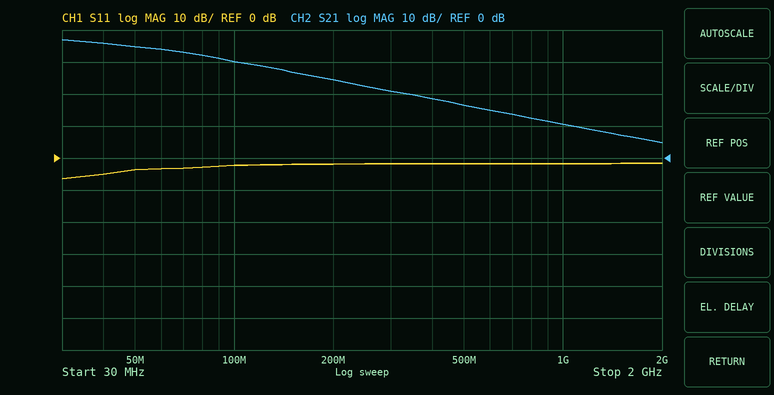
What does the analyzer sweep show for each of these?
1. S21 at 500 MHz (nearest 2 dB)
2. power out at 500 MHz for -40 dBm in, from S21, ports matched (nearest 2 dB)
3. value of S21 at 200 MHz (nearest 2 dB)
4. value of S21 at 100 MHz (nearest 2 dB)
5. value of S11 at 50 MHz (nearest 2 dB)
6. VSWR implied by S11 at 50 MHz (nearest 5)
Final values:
16 dB
-24 dBm
24 dB
30 dB
-4 dB
5
